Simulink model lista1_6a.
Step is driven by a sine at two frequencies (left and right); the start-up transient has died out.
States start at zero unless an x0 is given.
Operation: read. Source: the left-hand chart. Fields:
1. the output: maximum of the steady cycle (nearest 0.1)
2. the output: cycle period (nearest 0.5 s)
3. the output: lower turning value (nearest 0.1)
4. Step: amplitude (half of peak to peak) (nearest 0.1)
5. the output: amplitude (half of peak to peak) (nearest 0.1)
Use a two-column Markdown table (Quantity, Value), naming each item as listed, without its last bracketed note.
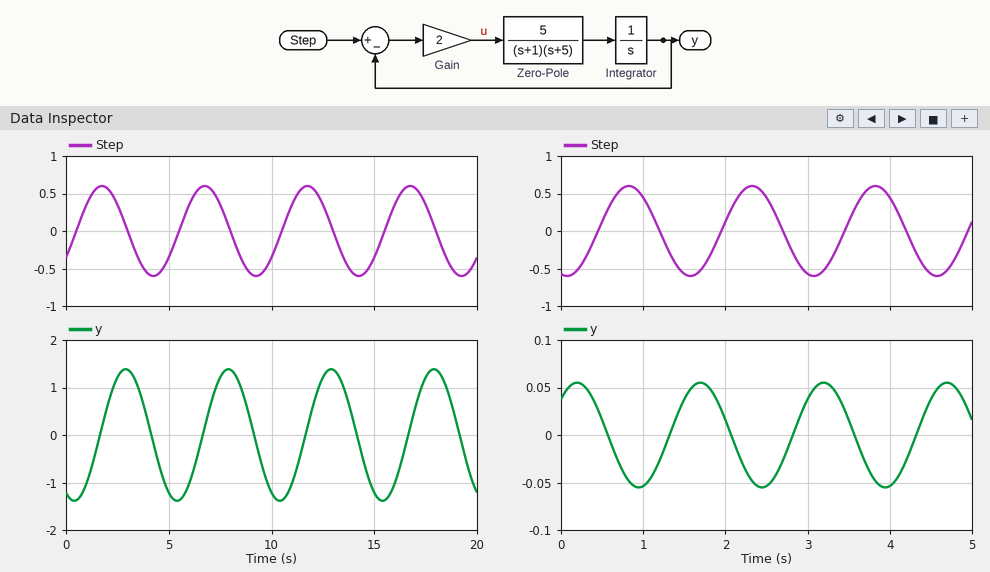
| Quantity | Value |
|---|---|
| the output: maximum of the steady cycle | 1.4 |
| the output: cycle period | 5.0 s |
| the output: lower turning value | -1.4 |
| Step: amplitude (half of peak to peak) | 0.6 |
| the output: amplitude (half of peak to peak) | 1.4 |
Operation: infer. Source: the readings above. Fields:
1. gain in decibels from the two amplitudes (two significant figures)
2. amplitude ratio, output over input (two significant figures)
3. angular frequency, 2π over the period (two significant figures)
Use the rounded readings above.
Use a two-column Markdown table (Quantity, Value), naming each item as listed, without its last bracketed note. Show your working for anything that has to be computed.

| Quantity | Value |
|---|---|
| gain in decibels from the two amplitudes | 20 log10(1.4 / 0.6) = 7.4 dB |
| amplitude ratio, output over input | 1.4 / 0.6 = 2.3 |
| angular frequency, 2π over the period | 2π / 5 = 1.3 rad/s |
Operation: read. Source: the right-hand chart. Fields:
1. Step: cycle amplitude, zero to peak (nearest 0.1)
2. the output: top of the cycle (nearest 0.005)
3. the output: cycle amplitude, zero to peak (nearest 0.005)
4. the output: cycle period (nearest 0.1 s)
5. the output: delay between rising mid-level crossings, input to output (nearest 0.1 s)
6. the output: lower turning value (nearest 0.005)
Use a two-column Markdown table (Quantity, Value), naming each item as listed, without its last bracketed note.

| Quantity | Value |
|---|---|
| Step: cycle amplitude, zero to peak | 0.6 |
| the output: top of the cycle | 0.055 |
| the output: cycle amplitude, zero to peak | 0.055 |
| the output: cycle period | 1.5 s |
| the output: delay between rising mid-level crossings, input to output | 0.9 s |
| the output: lower turning value | -0.055 |
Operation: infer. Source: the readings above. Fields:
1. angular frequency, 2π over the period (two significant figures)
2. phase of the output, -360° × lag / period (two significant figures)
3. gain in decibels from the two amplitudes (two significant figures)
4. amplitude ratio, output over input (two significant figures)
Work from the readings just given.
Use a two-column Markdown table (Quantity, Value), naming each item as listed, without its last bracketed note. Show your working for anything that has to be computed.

| Quantity | Value |
|---|---|
| angular frequency, 2π over the period | 2π / 1.5 = 4.2 rad/s |
| phase of the output, -360° × lag / period | -360 × 0.9 / 1.5 = -220° |
| gain in decibels from the two amplitudes | 20 log10(0.055 / 0.6) = -21 dB |
| amplitude ratio, output over input | 0.055 / 0.6 = 0.092 |
